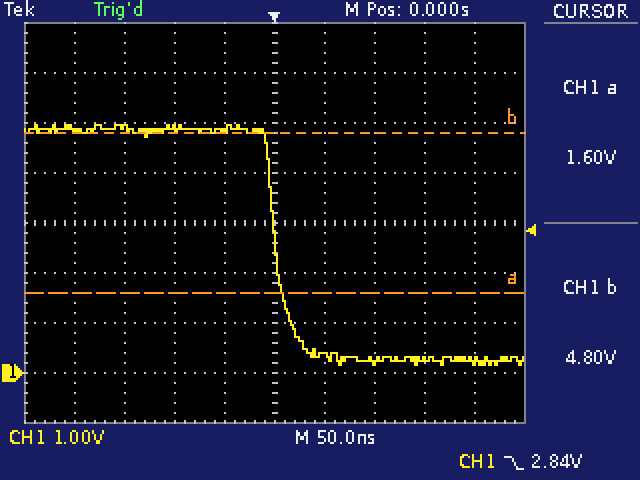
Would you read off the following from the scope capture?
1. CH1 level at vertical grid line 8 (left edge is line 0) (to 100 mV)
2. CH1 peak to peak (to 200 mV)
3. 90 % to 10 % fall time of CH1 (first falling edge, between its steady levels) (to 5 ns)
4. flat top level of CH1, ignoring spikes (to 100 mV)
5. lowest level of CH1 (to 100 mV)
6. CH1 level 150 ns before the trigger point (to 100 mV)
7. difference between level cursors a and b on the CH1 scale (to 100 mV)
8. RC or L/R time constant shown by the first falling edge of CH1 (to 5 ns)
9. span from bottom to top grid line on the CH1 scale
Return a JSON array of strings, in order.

["300 mV", "4.8 V", "30 ns", "4.9 V", "200 mV", "4.9 V", "3.2 V", "15 ns", "8 V"]
